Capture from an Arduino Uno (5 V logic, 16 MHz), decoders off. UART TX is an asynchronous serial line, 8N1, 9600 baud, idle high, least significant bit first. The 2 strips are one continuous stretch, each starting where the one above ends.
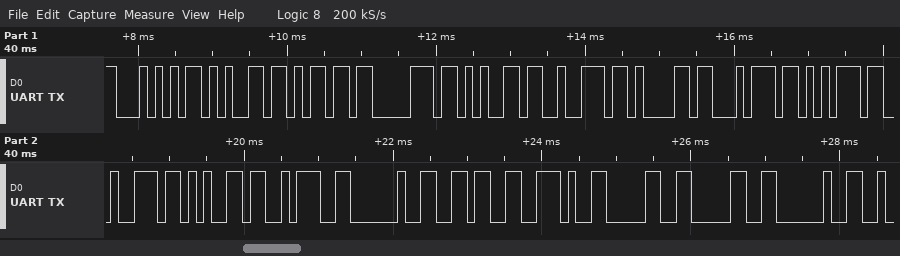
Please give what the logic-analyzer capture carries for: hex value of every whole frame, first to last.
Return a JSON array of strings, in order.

["54 65 6D 70 65 72 61 74 75 72 65 3A 20 36 2E 30 30 20"]
